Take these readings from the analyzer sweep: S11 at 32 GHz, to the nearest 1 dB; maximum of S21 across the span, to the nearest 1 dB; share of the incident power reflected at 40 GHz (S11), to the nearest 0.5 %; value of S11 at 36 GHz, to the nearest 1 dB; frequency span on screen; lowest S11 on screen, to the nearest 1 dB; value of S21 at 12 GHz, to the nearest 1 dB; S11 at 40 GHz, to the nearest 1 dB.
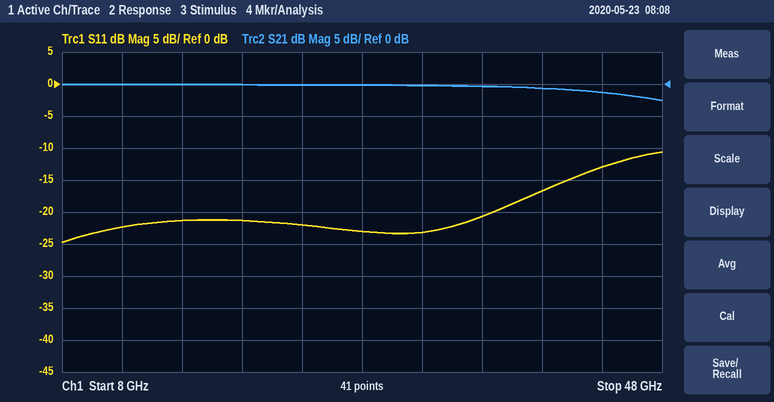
-23 dB
0 dB
2.0 %
-21 dB
40 GHz
-25 dB
0 dB
-17 dB
